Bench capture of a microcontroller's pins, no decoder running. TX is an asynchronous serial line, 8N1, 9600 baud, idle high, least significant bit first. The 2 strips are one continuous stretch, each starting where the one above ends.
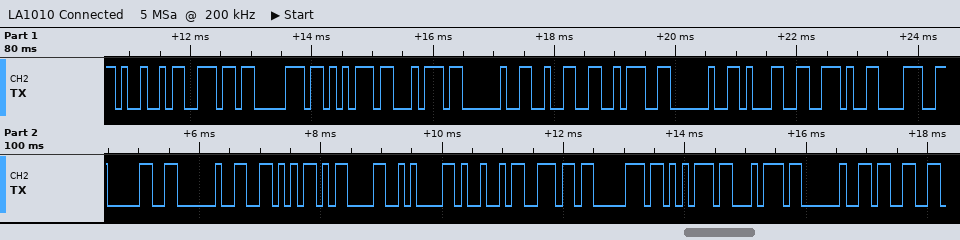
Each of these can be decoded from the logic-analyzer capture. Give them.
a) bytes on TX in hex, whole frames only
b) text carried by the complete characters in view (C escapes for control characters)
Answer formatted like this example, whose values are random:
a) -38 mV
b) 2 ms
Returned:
a) 0x49 0x6E 0x70 0x75 0x74 0x20 0x32 0x3A 0x20 0x31 0x2E 0x38 0x30 0x20 0x56 0x0D 0x0A 0x49 0x6E 0x70 0x75 0x74 0x20 0x33
b) "Input 2: 1.80 V\r\nInput 3"
